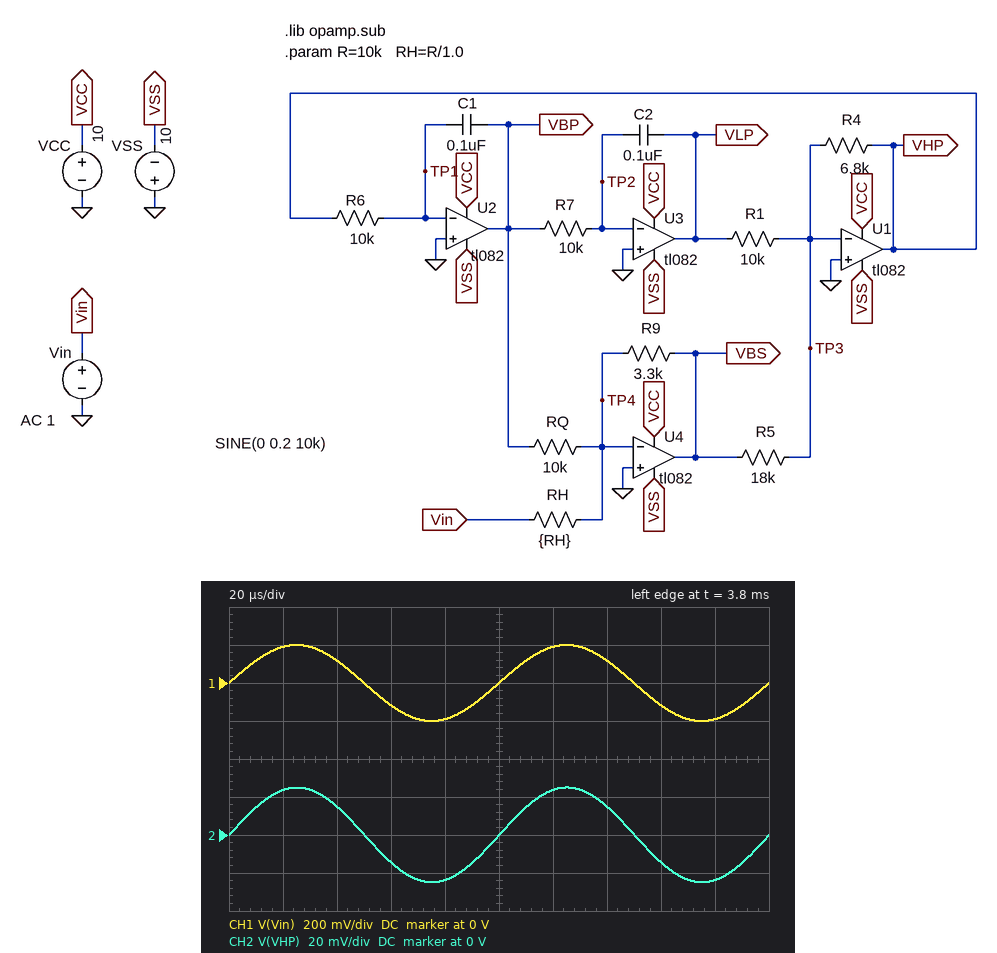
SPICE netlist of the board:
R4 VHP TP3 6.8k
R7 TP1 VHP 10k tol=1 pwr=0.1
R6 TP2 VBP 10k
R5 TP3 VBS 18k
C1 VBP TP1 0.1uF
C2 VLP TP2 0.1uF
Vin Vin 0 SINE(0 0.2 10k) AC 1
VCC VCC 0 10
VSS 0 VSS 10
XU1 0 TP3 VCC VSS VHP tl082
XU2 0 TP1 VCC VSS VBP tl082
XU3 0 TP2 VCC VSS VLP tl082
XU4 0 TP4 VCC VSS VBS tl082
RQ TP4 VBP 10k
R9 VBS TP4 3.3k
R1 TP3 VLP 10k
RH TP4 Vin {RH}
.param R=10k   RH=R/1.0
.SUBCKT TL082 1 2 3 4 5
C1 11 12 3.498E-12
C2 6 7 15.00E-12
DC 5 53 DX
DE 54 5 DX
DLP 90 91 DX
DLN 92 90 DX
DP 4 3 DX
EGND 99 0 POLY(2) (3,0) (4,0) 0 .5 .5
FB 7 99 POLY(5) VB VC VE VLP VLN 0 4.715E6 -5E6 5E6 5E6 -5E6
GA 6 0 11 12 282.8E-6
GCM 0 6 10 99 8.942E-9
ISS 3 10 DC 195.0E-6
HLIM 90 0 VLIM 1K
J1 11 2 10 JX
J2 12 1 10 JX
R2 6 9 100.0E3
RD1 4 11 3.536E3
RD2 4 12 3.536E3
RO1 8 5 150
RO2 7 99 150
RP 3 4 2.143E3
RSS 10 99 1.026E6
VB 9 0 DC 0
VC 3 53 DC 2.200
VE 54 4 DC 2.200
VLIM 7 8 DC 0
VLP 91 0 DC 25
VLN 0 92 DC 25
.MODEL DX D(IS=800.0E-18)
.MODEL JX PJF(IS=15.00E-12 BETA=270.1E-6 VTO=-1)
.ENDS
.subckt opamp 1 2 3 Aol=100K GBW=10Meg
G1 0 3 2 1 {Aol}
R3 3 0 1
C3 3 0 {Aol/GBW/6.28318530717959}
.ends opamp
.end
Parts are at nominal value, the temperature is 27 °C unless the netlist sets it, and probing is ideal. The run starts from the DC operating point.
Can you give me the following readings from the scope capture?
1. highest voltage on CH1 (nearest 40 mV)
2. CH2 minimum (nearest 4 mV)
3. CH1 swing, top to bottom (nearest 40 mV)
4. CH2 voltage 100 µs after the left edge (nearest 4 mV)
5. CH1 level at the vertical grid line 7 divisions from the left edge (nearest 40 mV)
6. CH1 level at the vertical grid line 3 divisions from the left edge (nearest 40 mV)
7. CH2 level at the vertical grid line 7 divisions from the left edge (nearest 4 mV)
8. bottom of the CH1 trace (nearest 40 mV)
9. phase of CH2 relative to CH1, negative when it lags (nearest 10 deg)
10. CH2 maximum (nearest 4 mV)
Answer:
200 mV
-24 mV
400 mV
0 V
120 mV
-120 mV
16 mV
-200 mV
0 deg
24 mV
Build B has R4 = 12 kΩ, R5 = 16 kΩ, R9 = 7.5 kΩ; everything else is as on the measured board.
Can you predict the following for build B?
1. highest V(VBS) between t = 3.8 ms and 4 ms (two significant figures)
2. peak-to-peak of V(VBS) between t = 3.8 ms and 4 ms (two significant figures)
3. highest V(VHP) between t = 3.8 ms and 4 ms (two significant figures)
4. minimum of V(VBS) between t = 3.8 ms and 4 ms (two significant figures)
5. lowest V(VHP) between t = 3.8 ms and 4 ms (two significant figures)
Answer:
150 mV
300 mV
110 mV
-150 mV
-110 mV
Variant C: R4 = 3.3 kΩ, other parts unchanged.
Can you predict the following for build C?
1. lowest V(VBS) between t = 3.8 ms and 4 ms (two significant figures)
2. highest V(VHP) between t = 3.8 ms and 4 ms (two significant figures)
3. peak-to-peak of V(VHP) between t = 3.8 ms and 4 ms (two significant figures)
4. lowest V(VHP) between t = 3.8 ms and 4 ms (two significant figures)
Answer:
-66 mV
12 mV
24 mV
-12 mV
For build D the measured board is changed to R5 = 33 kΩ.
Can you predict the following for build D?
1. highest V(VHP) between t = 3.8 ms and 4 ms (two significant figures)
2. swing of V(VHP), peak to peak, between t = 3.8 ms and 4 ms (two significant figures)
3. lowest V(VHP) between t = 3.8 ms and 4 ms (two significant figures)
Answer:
14 mV
27 mV
-14 mV
